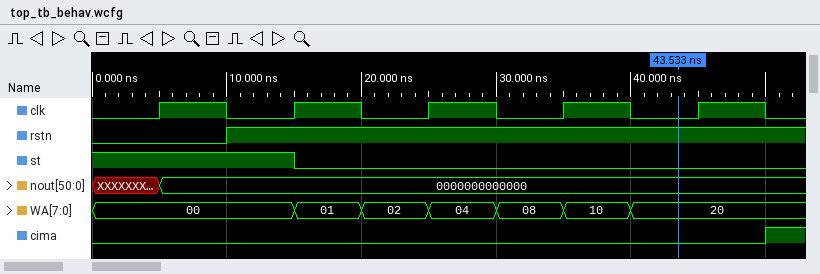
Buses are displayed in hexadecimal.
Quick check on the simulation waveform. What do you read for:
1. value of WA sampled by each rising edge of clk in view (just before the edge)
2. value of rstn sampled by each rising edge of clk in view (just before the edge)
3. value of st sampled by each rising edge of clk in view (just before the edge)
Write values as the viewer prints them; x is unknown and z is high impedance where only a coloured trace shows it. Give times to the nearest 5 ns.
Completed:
00, 00, 02, 08, 20
0 1 1 1 1
1 1 0 0 0
